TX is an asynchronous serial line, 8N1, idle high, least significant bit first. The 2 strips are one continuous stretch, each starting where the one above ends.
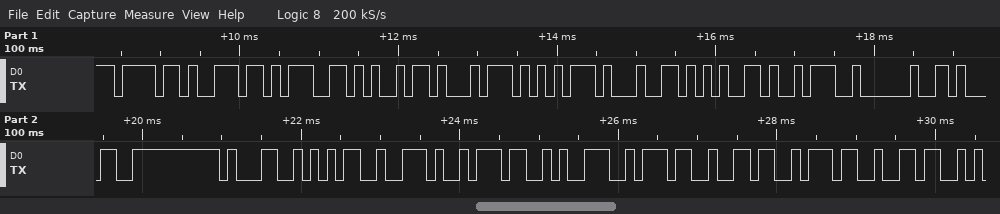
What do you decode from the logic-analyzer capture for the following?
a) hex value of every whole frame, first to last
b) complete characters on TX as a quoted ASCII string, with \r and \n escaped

6F 6E 67 69 74 75 64 65 3A 20 31 31 35 2E 37 39 37 36 37 36
"ongitude: 115.797676"
